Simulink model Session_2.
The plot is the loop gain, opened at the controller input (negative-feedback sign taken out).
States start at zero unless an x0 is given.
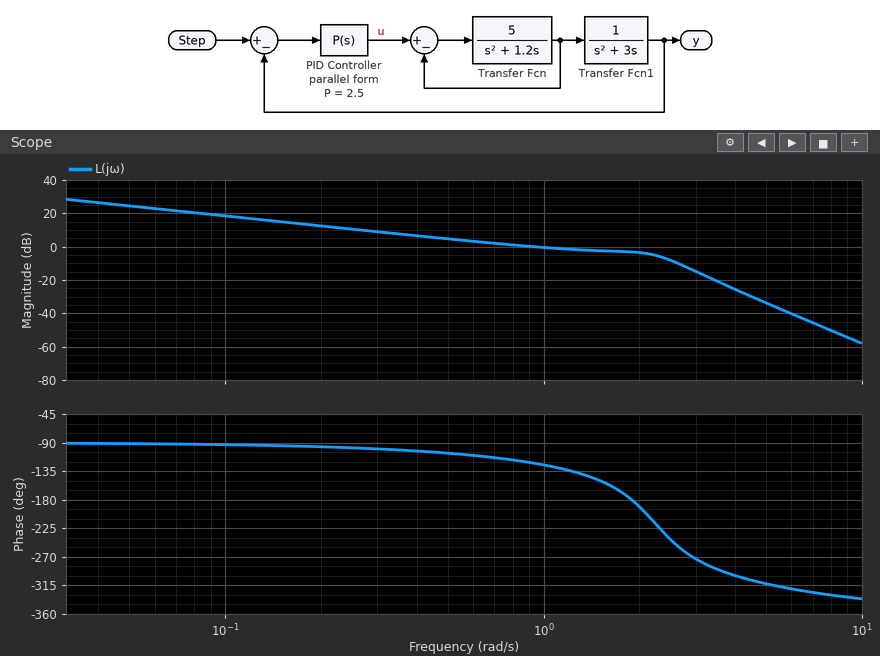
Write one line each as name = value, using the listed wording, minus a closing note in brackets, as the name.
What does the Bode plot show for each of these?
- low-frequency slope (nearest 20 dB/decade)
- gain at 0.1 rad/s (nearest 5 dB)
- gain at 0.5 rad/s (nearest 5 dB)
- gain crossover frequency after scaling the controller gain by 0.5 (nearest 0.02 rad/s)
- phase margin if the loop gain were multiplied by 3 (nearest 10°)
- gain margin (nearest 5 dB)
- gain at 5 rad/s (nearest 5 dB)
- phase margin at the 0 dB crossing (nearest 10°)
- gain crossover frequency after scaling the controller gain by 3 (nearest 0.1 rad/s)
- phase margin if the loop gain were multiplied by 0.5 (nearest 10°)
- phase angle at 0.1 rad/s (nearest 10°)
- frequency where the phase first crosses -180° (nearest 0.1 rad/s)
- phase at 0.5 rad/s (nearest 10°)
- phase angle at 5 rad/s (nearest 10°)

low-frequency slope = -20 dB/decade
gain at 0.1 rad/s = 20 dB
gain at 0.5 rad/s = 5 dB
gain crossover frequency after scaling the controller gain by 0.5 = 0.42 rad/s
phase margin if the loop gain were multiplied by 3 = -70°
gain margin = 5 dB
gain at 5 rad/s = -35 dB
phase margin at the 0 dB crossing = 60°
gain crossover frequency after scaling the controller gain by 3 = 2.6 rad/s
phase margin if the loop gain were multiplied by 0.5 = 80°
phase angle at 0.1 rad/s = -90°
frequency where the phase first crosses -180° = 1.9 rad/s
phase at 0.5 rad/s = -110°
phase angle at 5 rad/s = -310°
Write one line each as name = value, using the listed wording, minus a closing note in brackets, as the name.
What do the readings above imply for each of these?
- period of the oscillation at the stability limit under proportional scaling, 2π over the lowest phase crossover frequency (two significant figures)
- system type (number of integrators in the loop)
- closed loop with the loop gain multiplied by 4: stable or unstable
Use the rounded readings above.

period of the oscillation at the stability limit under proportional scaling, 2π over the lowest phase crossover frequency = 3.3 s
system type = 1
closed loop with the loop gain multiplied by 4: stable or unstable = unstable
